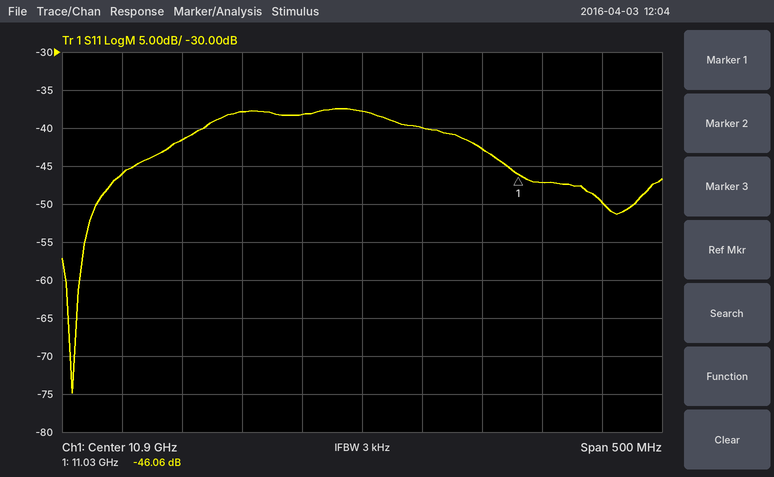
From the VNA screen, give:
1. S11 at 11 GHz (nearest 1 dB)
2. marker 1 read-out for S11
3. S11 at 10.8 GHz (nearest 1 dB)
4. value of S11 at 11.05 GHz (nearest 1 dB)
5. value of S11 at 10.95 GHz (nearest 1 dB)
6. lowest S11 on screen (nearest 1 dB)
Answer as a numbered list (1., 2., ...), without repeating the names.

1. -43 dB
2. -46.06 dB
3. -38 dB
4. -47 dB
5. -40 dB
6. -75 dB
